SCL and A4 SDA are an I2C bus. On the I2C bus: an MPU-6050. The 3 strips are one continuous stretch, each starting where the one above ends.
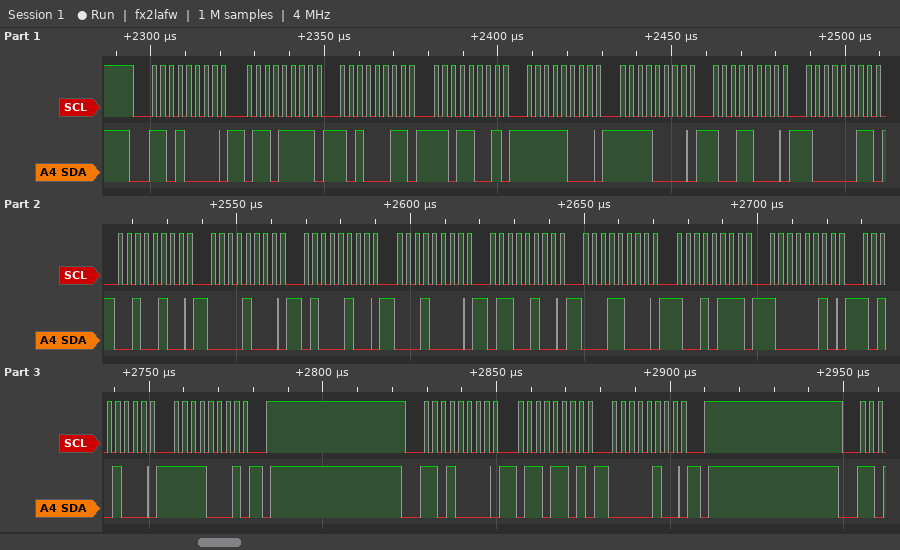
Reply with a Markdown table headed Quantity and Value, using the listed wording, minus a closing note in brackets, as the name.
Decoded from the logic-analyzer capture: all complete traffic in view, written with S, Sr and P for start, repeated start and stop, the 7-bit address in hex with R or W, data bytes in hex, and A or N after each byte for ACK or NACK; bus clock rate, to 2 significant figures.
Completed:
| Quantity | Value |
|---|---|
| all complete traffic in view, written with S, Sr and P for start, repeated start and stop, the 7-bit address in hex with R or W, data bytes in hex, and A or N after each byte for ACK or NACK | S 68W A 6F A A3 A D9 A F8 A F0 A 98 A 83 A 24 A 08 A 44 A 10 A 64 A 18 A 97 A 82 A A8 A F1 A P S 68W A 6D A 04 A P |
| bus clock rate, to 2 significant figures | 400 kHz |
